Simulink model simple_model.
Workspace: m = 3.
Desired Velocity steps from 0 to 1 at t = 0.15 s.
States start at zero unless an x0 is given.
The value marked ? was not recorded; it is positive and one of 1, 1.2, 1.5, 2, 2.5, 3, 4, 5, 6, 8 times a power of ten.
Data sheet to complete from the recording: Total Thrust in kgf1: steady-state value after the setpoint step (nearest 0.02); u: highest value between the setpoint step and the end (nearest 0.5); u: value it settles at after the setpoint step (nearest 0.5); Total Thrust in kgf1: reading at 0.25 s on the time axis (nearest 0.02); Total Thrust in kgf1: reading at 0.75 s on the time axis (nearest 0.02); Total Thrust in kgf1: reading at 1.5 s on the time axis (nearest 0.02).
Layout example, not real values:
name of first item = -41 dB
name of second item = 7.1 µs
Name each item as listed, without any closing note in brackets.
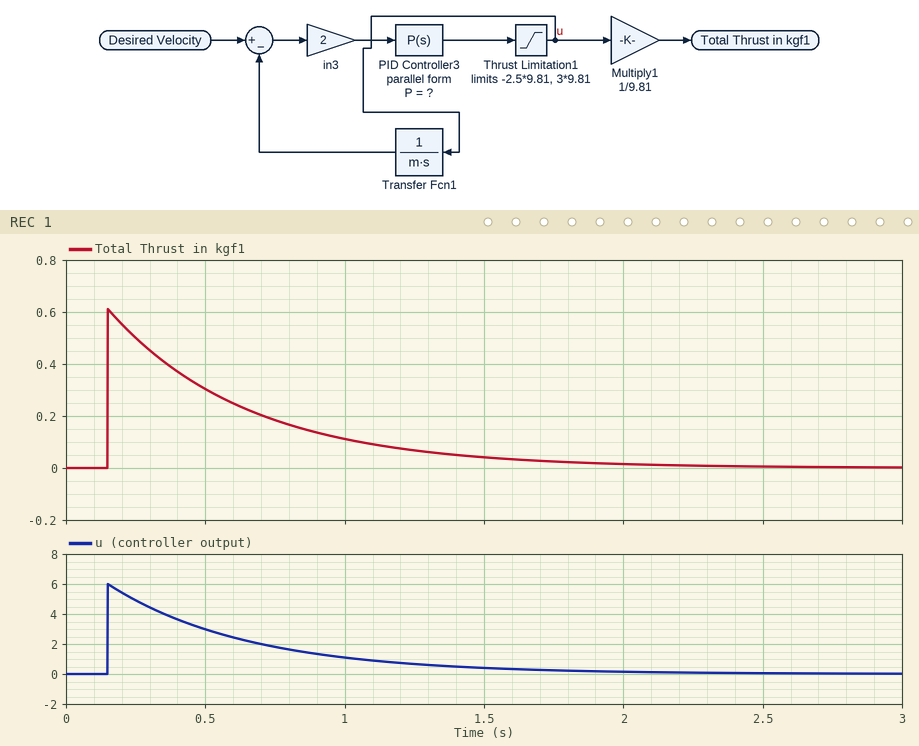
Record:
Total Thrust in kgf1: steady-state value after the setpoint step = 0.00
u: highest value between the setpoint step and the end = 6.0
u: value it settles at after the setpoint step = 0.0
Total Thrust in kgf1: reading at 0.25 s on the time axis = 0.50
Total Thrust in kgf1: reading at 0.75 s on the time axis = 0.18
Total Thrust in kgf1: reading at 1.5 s on the time axis = 0.04
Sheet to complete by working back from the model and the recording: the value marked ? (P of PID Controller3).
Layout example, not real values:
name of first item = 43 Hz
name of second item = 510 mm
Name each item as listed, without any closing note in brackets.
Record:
the value marked ? = 3
